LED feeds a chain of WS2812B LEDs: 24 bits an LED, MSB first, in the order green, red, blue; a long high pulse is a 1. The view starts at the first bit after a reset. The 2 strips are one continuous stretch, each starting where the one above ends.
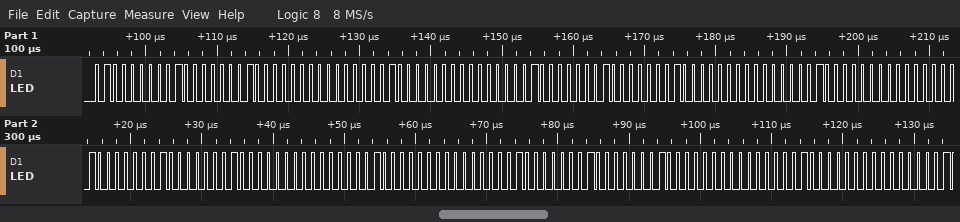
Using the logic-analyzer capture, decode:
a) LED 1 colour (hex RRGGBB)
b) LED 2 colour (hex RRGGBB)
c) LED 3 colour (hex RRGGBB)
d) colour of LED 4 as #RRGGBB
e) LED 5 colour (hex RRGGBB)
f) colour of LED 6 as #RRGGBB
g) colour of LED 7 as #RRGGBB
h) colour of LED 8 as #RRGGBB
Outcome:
#404040
#400000
#404040
#400000
#404040
#400000
#404040
#400000
